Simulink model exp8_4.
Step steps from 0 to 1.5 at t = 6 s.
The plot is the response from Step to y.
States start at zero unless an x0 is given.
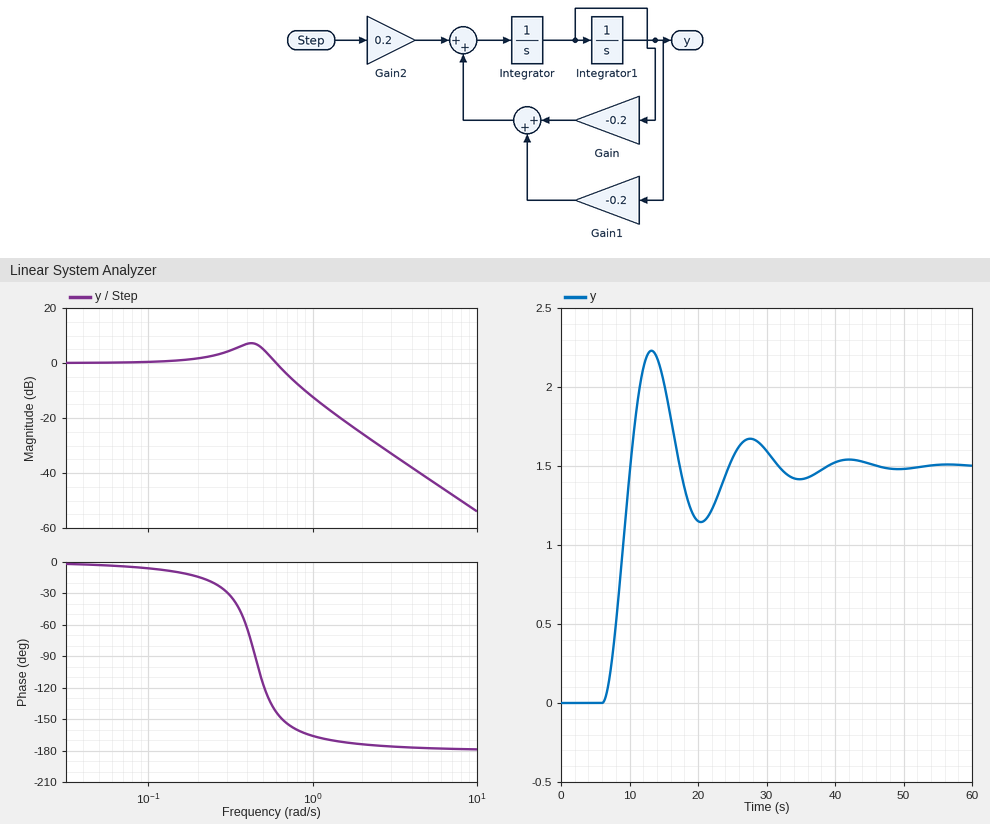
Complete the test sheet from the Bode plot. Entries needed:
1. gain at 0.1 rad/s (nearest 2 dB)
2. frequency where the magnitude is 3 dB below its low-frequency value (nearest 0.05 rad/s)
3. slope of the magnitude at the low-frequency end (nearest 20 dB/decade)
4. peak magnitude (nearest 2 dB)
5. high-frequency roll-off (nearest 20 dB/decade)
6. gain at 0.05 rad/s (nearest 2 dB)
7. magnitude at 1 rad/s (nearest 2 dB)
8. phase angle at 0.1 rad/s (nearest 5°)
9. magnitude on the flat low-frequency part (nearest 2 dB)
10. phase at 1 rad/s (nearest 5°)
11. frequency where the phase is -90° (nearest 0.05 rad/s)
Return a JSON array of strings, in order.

["0 dB", "0.65 rad/s", "0 dB/decade", "8 dB", "-40 dB/decade", "0 dB", "-12 dB", "-5°", "0 dB", "-165°", "0.45 rad/s"]
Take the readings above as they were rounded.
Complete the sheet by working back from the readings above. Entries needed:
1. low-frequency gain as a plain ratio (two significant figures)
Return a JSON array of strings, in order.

["1.0"]
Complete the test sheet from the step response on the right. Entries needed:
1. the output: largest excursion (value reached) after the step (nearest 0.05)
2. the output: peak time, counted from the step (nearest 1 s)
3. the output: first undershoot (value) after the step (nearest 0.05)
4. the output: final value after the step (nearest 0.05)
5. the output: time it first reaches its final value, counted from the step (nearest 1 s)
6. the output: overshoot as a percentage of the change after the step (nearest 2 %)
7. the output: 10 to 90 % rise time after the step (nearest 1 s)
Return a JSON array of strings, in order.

["2.25", "7 s", "1.15", "1.50", "4 s", "48 %", "3 s"]
